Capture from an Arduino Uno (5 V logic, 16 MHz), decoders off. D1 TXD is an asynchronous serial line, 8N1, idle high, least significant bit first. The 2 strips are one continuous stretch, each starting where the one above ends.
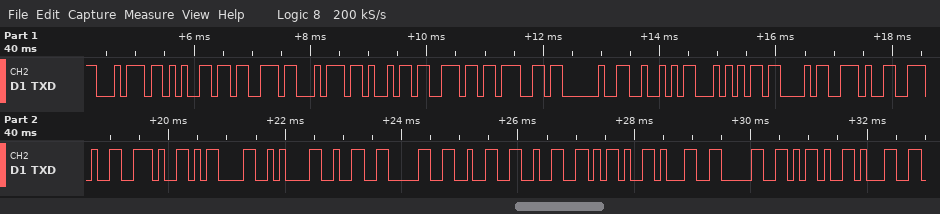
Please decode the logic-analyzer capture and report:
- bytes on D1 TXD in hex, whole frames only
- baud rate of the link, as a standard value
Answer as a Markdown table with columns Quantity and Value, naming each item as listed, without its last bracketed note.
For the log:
| Quantity | Value |
|---|---|
| bytes on D1 TXD in hex, whole frames only | 74 65 73 74 69 6E 67 20 52 54 43 2E 2E 2E 0D 0A 32 30 32 32 2D 31 30 2D 31 |
| baud rate of the link, as a standard value | 9600 baud |
